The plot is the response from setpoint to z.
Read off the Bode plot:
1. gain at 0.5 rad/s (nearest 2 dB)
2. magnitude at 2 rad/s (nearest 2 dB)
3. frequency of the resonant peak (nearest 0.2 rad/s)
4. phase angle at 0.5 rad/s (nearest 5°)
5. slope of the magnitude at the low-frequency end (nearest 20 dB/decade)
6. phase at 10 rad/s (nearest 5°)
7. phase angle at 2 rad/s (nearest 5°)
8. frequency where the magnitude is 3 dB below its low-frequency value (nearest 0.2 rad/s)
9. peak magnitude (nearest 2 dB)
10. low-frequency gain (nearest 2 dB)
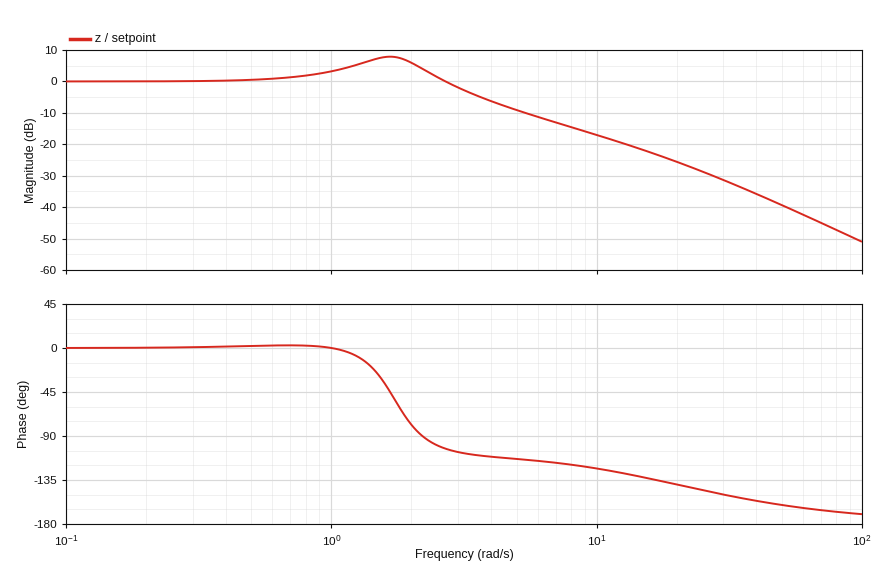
0 dB
6 dB
1.6 rad/s
0°
0 dB/decade
-125°
-80°
3.2 rad/s
8 dB
0 dB
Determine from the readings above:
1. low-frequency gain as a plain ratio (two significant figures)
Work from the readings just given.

1.0
